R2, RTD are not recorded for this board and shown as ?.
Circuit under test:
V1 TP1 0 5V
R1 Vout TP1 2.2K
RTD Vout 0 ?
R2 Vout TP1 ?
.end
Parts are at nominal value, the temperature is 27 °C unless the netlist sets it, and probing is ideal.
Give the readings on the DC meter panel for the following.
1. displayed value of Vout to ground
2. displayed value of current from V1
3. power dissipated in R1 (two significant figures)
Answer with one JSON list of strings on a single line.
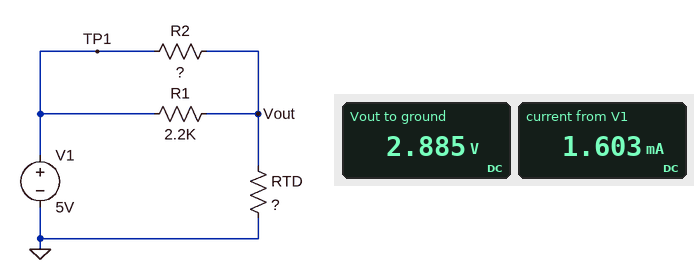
["2.885 V", "1.603 mA", "2.0 mW"]
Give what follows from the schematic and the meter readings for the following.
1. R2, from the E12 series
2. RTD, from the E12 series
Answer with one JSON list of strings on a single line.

["3.3 kΩ", "1.8 kΩ"]
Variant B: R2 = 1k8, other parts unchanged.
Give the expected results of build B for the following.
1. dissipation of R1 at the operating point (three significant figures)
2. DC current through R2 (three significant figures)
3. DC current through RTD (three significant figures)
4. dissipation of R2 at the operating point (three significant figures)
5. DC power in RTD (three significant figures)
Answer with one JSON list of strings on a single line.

["1.43 mW", "986 µA", "1.79 mA", "1.75 mW", "5.78 mW"]
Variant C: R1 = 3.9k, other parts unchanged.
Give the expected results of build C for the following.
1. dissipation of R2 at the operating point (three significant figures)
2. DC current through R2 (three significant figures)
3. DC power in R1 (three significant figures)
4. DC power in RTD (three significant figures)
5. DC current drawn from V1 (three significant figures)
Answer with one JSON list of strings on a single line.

["1.88 mW", "755 µA", "1.59 mW", "3.50 mW", "1.39 mA"]
